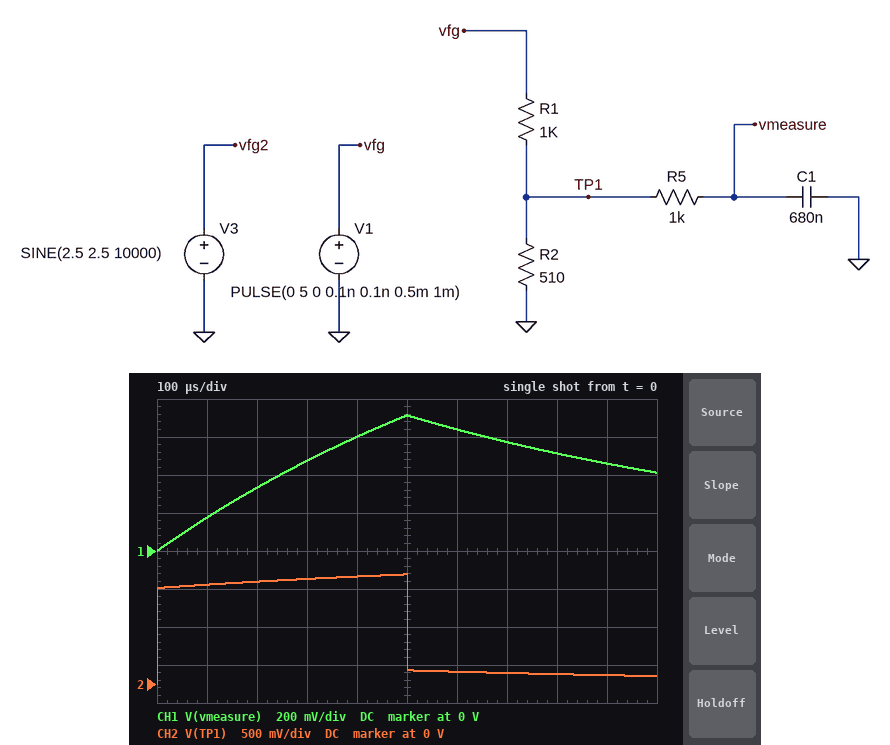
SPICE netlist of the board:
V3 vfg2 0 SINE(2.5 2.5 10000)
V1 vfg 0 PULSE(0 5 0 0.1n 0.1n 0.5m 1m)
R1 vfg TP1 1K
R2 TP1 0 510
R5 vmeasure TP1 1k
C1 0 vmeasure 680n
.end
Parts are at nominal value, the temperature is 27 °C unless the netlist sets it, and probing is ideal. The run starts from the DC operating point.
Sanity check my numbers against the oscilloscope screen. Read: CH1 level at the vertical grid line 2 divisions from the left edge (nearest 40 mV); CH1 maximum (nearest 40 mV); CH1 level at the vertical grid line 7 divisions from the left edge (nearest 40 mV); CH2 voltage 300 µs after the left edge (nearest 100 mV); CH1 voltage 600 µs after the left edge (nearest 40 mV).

320 mV
720 mV
560 mV
1.4 V
640 mV
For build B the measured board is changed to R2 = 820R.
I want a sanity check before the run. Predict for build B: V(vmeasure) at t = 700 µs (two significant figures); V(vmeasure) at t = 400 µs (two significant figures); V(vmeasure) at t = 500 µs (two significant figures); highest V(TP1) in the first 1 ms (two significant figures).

730 mV
750 mV
900 mV
1.8 V
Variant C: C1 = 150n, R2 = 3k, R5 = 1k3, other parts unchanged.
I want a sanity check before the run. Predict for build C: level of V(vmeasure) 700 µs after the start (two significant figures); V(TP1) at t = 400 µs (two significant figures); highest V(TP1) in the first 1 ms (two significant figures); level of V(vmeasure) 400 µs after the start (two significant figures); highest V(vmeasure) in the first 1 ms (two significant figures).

1.6 V
3.4 V
3.5 V
2.7 V
3.0 V
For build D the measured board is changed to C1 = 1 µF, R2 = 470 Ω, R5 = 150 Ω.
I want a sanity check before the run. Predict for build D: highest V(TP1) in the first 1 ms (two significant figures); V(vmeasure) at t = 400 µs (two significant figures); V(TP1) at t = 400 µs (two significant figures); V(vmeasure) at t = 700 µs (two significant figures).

1.2 V
920 mV
1.1 V
680 mV
